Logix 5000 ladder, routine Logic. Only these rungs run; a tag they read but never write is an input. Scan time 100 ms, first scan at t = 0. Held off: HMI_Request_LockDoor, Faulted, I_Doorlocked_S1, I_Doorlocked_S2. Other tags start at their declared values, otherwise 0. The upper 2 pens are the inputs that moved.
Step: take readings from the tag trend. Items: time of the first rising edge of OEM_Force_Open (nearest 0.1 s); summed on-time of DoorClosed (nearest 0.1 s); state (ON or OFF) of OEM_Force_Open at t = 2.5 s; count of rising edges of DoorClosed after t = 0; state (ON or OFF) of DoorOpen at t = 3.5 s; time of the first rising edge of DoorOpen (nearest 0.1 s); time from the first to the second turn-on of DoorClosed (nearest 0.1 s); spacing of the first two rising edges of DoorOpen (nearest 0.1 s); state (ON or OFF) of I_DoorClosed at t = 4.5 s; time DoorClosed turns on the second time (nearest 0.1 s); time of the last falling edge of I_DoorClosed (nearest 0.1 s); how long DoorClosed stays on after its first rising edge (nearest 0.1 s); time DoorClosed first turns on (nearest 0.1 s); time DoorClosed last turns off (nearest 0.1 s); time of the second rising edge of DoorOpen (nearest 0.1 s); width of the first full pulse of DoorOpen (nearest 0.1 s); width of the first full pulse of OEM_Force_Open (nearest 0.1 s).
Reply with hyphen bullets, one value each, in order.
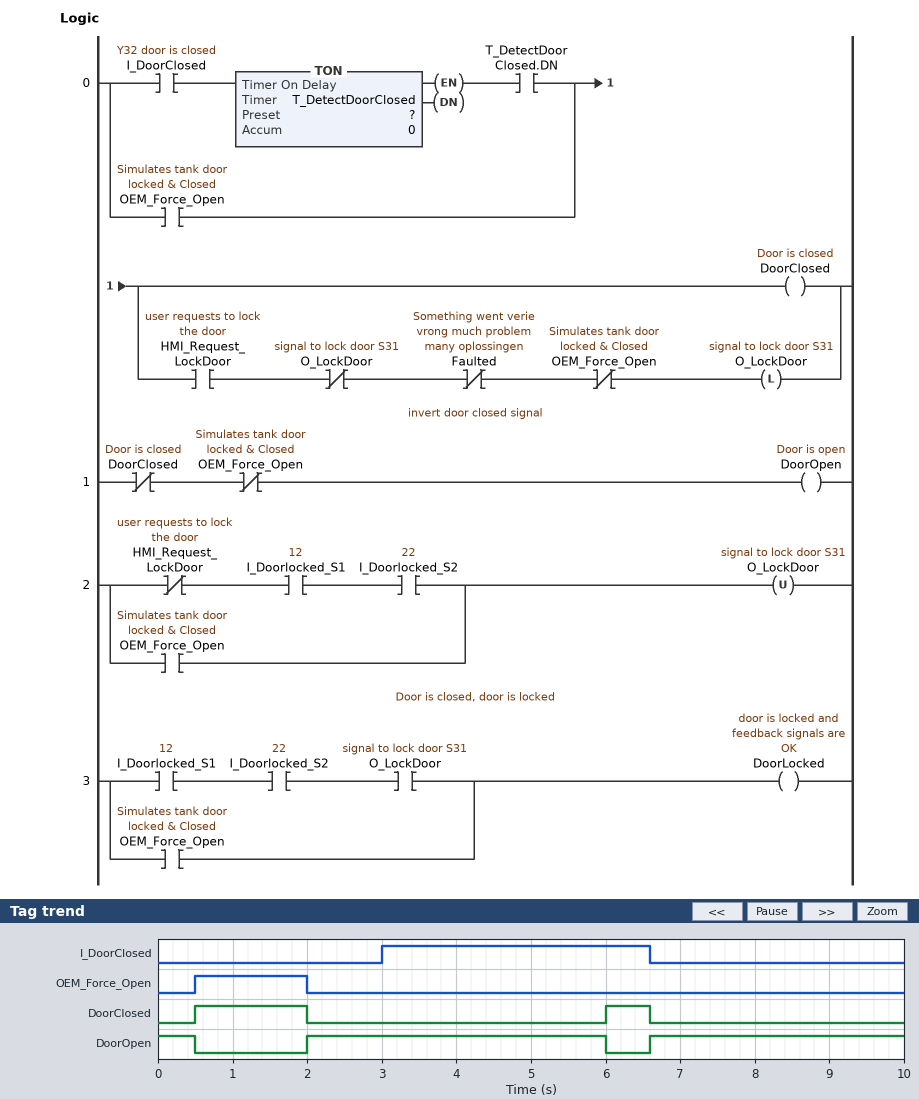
- 0.5 s
- 2.1 s
- OFF
- 2
- ON
- 2.0 s
- 5.5 s
- 4.6 s
- ON
- 6.0 s
- 6.6 s
- 1.5 s
- 0.5 s
- 6.6 s
- 6.6 s
- 4.0 s
- 1.5 s
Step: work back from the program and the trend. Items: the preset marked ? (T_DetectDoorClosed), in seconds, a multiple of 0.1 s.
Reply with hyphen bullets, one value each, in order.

- 3.0 s
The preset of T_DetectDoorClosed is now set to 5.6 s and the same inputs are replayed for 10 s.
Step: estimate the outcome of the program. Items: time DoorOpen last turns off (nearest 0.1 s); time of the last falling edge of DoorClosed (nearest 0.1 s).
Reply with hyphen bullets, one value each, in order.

- 0.5 s
- 2.0 s
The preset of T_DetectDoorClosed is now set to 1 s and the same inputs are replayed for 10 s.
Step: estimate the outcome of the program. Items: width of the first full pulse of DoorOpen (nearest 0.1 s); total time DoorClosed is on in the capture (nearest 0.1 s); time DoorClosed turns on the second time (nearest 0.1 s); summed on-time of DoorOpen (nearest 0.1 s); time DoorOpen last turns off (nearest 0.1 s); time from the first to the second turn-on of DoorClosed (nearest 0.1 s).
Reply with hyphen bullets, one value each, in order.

- 2.0 s
- 4.1 s
- 4.0 s
- 5.9 s
- 4.0 s
- 3.5 s
